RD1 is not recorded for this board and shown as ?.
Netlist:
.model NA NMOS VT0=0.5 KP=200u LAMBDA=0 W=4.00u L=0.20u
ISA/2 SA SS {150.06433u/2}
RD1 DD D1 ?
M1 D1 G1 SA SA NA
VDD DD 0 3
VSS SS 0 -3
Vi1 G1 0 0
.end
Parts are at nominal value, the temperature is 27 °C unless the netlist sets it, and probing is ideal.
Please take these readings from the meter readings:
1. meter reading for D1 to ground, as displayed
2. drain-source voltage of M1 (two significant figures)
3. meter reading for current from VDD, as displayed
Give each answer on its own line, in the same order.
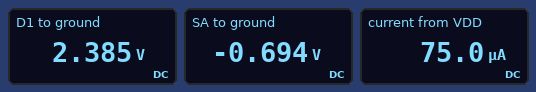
2.385 V
3.1 V
75.0 µA
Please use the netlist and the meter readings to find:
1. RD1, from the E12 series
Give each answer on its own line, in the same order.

8.2 kΩ
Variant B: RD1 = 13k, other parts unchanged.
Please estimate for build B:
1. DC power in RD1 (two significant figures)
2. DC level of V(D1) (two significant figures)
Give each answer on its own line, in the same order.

73 µW
2.0 V
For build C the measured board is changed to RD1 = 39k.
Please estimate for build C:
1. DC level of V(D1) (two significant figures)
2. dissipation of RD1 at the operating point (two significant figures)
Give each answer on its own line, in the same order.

74 mV
220 µW
